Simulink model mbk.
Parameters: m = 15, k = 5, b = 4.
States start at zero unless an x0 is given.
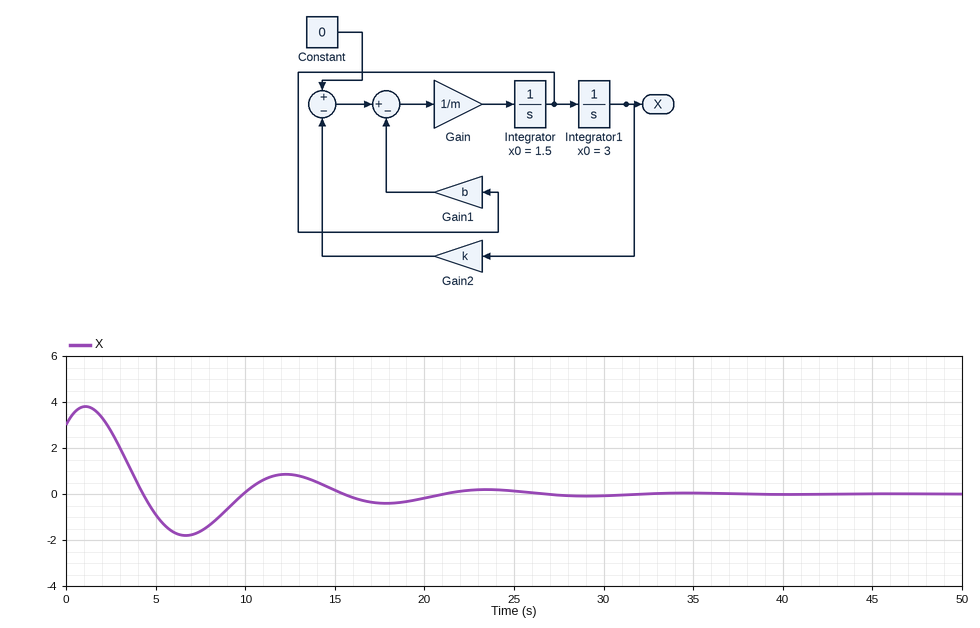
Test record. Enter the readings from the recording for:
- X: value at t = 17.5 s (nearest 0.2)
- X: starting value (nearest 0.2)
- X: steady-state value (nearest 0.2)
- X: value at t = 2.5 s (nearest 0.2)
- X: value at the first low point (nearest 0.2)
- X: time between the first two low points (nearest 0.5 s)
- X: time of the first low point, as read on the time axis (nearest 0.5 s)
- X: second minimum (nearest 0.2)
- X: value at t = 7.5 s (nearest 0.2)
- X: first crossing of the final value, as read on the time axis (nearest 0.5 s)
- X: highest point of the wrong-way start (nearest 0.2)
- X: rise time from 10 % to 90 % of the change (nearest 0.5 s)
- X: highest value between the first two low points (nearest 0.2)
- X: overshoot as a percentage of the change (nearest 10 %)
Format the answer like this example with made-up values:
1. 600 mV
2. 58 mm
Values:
1. -0.4
2. 3.0
3. 0.0
4. 2.8
5. -1.8
6. 11.0 s
7. 6.5 s
8. -0.4
9. -1.6
10. 4.5 s
11. 3.8
12. 1.5 s
13. 0.8
14. 60 %
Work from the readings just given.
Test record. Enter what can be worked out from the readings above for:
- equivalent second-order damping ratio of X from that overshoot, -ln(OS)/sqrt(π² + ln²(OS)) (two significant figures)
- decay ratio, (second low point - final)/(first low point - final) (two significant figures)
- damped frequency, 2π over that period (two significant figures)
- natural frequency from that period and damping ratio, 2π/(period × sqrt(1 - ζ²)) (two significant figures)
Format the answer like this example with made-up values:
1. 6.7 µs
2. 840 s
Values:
1. 0.16
2. 0.22
3. 0.57 rad/s
4. 0.58 rad/s
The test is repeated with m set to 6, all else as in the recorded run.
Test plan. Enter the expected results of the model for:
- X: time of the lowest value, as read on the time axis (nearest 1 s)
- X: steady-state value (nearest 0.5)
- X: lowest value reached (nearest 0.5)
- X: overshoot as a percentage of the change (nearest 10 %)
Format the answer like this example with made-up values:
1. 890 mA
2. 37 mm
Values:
1. 4 s
2. 0.0
3. -1.0
4. 30 %
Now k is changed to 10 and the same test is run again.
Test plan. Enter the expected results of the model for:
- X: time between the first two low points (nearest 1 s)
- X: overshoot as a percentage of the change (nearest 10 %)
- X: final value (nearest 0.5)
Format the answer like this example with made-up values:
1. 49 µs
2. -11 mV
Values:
1. 8 s
2. 70 %
3. 0.0
